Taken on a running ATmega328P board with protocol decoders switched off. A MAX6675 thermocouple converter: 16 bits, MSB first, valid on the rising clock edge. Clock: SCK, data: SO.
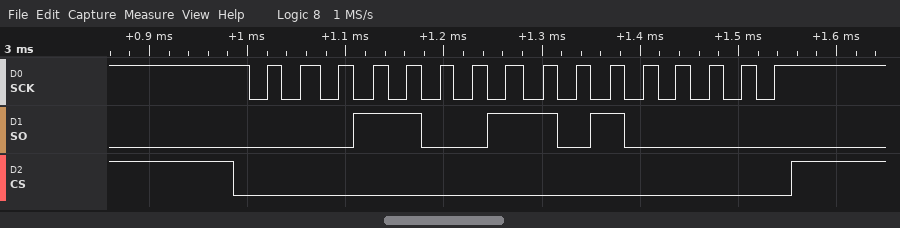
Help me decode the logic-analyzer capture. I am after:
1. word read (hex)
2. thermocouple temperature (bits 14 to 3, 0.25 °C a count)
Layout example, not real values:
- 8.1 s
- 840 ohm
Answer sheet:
- 0x19A0
- 205.00 °C
